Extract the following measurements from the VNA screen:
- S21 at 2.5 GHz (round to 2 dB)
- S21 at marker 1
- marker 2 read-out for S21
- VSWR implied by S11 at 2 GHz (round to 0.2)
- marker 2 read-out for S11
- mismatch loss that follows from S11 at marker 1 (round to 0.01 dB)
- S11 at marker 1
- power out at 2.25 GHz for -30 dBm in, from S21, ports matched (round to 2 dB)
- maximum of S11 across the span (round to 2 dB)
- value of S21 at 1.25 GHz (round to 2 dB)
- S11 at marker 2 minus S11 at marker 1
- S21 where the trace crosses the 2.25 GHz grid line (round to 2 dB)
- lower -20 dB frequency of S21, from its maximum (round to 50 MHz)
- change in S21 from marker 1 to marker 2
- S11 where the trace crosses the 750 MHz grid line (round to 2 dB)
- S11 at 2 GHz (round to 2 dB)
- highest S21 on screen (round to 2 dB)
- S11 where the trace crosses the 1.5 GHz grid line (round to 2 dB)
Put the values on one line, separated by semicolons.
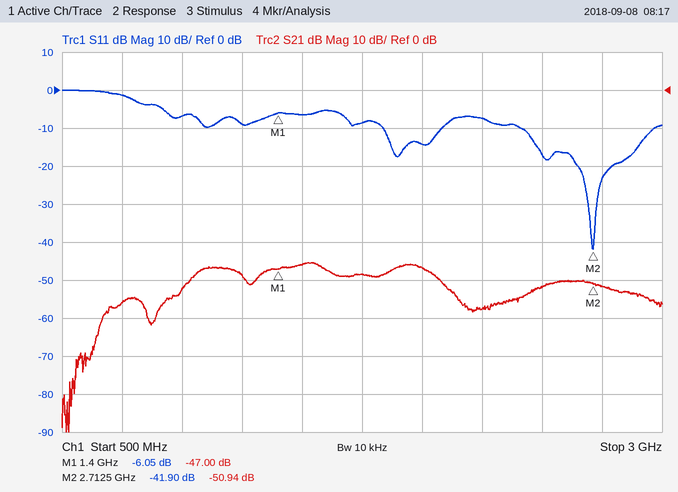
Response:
-52 dB; -47.00 dB; -50.94 dB; 1.4; -41.90 dB; 1.24 dB; -6.05 dB; -88 dBm; 0 dB; -48 dB; -35.85 dB; -58 dB; 650 MHz; -3.94 dB; -2 dB; -14 dB; -46 dB; -6 dB
